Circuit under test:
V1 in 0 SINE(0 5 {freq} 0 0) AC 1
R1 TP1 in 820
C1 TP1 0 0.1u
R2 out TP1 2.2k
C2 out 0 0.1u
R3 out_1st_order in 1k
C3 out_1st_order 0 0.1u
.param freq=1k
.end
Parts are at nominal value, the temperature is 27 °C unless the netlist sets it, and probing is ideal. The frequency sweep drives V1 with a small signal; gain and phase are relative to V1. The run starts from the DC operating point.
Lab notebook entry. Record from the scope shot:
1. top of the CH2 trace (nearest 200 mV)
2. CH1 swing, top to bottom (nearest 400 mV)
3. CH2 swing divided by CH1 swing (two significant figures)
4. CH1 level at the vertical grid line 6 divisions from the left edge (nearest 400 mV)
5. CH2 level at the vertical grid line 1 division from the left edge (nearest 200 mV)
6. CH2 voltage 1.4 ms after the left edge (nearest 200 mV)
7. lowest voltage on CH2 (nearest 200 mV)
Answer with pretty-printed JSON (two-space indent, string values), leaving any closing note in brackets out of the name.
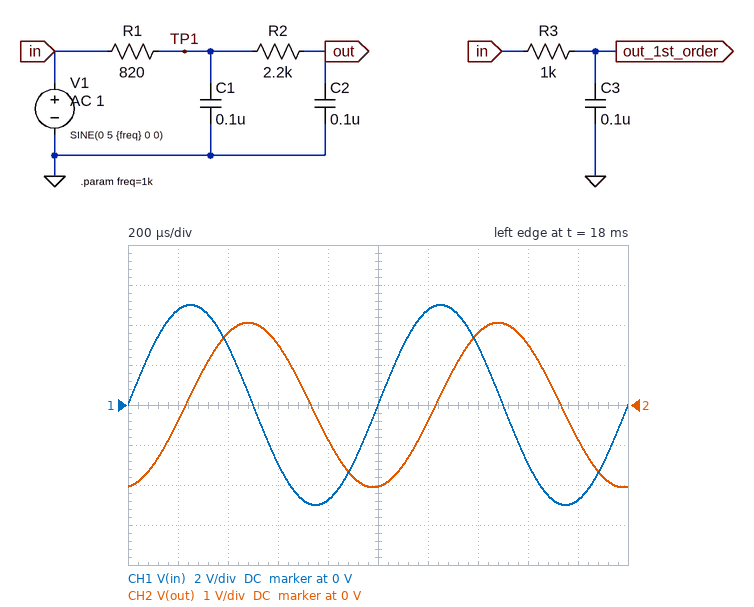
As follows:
{
  "top of the CH2 trace": "2.0 V",
  "CH1 swing, top to bottom": "10.0 V",
  "CH2 swing divided by CH1 swing": "0.41",
  "CH1 level at the vertical grid line 6 divisions from the left edge": "4.8 V",
  "CH2 level at the vertical grid line 1 division from the left edge": "-400 mV",
  "CH2 voltage 1.4 ms after the left edge": "1.8 V",
  "lowest voltage on CH2": "-2.0 V"
}
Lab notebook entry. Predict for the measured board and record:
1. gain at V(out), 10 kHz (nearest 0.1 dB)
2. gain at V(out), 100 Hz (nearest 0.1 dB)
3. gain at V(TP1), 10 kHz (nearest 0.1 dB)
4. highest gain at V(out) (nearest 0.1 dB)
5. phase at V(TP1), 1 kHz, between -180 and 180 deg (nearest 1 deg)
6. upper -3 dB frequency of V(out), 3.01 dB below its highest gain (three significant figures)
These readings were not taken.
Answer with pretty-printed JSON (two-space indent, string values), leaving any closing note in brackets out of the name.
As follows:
{
  "gain at V(out), 10 kHz": "-37.4 dB",
  "gain at V(out), 100 Hz": "-0.2 dB",
  "gain at V(TP1), 10 kHz": "-14.6 dB",
  "highest gain at V(out)": "0 dB",
  "phase at V(TP1), 1 kHz, between -180 and 180 deg": "-29 deg",
  "upper -3 dB frequency of V(out), 3.01 dB below its highest gain": "471 Hz"
}
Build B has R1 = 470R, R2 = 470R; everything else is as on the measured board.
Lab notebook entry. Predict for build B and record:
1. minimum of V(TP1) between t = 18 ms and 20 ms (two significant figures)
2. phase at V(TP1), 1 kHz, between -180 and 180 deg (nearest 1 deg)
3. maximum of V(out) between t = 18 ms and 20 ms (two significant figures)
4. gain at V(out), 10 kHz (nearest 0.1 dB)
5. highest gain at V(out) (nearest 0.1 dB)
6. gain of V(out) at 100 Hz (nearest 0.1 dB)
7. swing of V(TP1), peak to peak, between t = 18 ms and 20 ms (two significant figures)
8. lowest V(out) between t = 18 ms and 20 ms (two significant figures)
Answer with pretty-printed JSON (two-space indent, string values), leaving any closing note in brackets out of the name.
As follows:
{
  "minimum of V(TP1) between t = 18 ms and 20 ms": "-4.1 V",
  "phase at V(TP1), 1 kHz, between -180 and 180 deg": "-28 deg",
  "maximum of V(out) between t = 18 ms and 20 ms": "3.9 V",
  "gain at V(out), 10 kHz": "-21.4 dB",
  "highest gain at V(out)": "0 dB",
  "gain of V(out) at 100 Hz": "0 dB",
  "swing of V(TP1), peak to peak, between t = 18 ms and 20 ms": "8.2 V",
  "lowest V(out) between t = 18 ms and 20 ms": "-3.9 V"
}
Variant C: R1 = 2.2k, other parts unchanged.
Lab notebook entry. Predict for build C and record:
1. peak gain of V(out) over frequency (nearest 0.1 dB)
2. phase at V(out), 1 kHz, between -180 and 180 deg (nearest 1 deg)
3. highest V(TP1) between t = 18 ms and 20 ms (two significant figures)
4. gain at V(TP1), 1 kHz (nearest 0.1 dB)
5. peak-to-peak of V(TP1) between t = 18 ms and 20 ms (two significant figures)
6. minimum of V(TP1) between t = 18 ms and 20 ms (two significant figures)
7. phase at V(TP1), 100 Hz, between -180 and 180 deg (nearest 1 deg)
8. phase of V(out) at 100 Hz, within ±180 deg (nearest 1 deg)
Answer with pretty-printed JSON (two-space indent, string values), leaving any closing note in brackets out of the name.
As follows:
{
  "peak gain of V(out) over frequency": "0 dB",
  "phase at V(out), 1 kHz, between -180 and 180 deg": "-102 deg",
  "highest V(TP1) between t = 18 ms and 20 ms": "2.0 V",
  "gain at V(TP1), 1 kHz": "-7.9 dB",
  "peak-to-peak of V(TP1) between t = 18 ms and 20 ms": "4.0 V",
  "minimum of V(TP1) between t = 18 ms and 20 ms": "-2.0 V",
  "phase at V(TP1), 100 Hz, between -180 and 180 deg": "-15 deg",
  "phase of V(out) at 100 Hz, within ±180 deg": "-23 deg"
}
